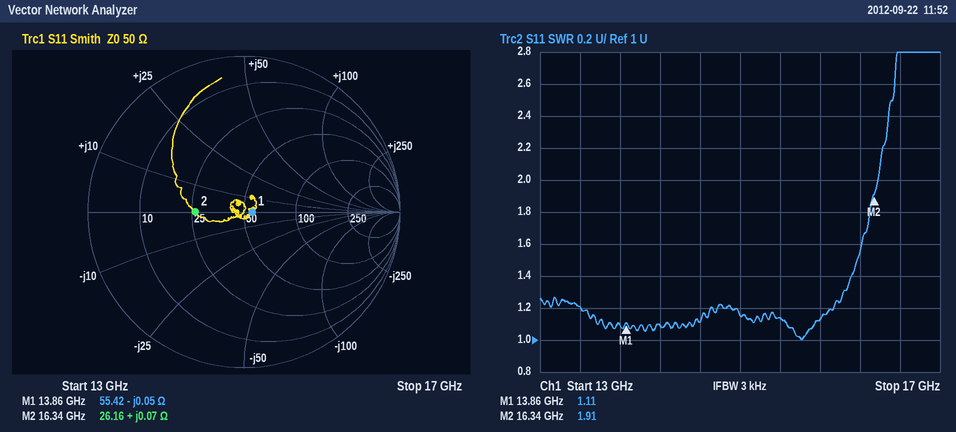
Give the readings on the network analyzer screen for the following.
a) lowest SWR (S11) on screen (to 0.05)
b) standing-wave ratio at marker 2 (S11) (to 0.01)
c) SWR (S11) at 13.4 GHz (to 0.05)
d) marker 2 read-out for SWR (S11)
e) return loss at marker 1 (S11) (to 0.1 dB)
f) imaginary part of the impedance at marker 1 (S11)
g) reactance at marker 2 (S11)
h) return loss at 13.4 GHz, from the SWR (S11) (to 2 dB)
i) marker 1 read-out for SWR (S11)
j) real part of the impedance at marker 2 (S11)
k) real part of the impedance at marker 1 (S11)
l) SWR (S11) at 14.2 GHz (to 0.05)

1.00
1.91
1.20
1.91
25.8 dB
-0.05 Ω
+0.07 Ω
20 dB
1.11
26.16 Ω
55.42 Ω
1.10
